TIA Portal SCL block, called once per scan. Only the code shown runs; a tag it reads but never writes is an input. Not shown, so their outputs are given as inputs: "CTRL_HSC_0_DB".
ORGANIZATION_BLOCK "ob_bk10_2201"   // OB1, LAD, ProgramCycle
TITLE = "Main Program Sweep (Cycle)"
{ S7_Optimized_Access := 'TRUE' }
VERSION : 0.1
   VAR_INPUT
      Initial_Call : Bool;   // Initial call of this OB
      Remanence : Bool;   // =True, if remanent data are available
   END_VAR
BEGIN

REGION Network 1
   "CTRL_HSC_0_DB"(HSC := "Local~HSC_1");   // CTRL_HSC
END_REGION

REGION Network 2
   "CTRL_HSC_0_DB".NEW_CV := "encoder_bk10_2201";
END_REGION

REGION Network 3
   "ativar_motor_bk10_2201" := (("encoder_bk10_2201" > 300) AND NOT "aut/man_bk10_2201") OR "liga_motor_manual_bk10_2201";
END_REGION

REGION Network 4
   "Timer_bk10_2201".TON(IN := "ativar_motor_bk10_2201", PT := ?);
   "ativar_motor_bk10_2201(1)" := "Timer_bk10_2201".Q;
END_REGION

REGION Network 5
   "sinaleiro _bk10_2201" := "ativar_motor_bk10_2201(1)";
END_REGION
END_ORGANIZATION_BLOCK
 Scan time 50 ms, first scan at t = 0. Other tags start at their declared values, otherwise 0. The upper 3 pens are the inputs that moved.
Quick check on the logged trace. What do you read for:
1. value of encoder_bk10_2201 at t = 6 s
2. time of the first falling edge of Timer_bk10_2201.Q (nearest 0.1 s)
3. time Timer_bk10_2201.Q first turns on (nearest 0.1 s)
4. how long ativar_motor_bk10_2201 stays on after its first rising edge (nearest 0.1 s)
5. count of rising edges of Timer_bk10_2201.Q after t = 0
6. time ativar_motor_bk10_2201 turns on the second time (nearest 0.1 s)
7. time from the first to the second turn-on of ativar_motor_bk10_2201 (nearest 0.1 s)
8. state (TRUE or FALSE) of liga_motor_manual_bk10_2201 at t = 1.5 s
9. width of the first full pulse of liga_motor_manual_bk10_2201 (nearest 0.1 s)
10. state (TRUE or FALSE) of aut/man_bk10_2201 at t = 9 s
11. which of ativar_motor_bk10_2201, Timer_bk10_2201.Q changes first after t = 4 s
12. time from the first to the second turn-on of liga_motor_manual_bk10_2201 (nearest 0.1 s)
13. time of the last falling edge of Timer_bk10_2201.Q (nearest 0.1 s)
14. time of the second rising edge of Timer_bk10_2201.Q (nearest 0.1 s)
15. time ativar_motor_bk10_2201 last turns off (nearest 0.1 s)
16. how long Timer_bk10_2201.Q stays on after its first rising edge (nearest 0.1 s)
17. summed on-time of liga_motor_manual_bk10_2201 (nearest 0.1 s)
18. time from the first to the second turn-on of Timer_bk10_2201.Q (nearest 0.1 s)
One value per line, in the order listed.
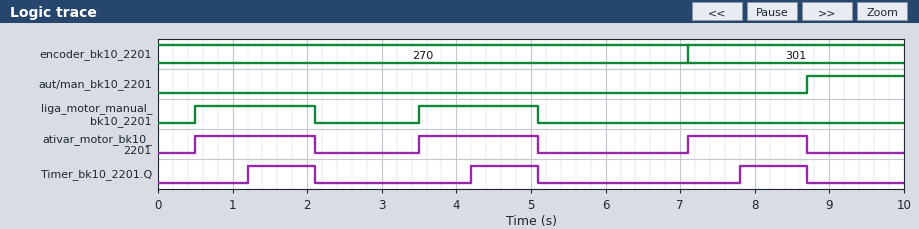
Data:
270
2.1 s
1.2 s
1.6 s
3
3.5 s
3.0 s
TRUE
1.6 s
TRUE
Timer_bk10_2201.Q
3.0 s
8.7 s
4.2 s
8.7 s
0.9 s
3.2 s
3.0 s
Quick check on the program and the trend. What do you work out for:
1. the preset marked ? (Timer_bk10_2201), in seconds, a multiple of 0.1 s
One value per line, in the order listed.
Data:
0.7 s
